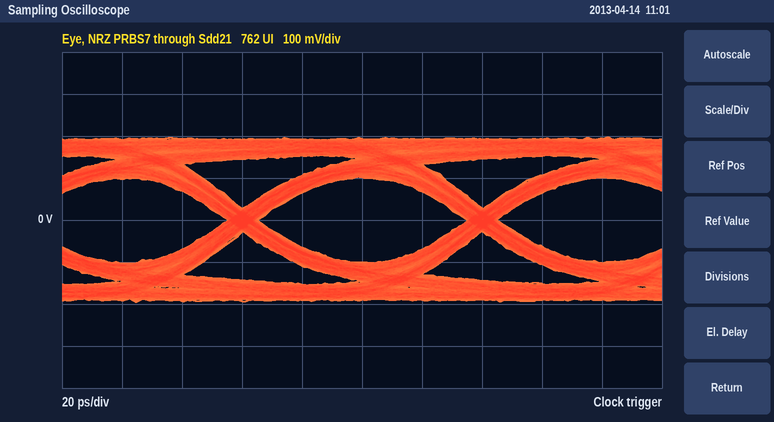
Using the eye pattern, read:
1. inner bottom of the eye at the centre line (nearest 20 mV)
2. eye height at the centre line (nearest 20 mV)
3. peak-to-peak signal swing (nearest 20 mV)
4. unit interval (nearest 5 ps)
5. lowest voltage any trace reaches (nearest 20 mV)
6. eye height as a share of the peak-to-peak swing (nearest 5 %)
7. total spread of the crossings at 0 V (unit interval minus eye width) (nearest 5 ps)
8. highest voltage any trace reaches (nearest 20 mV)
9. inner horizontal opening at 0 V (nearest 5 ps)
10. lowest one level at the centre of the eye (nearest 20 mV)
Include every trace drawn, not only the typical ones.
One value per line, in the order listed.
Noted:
-100 mV
200 mV
400 mV
80 ps
-200 mV
50 %
10 ps
200 mV
70 ps
100 mV
